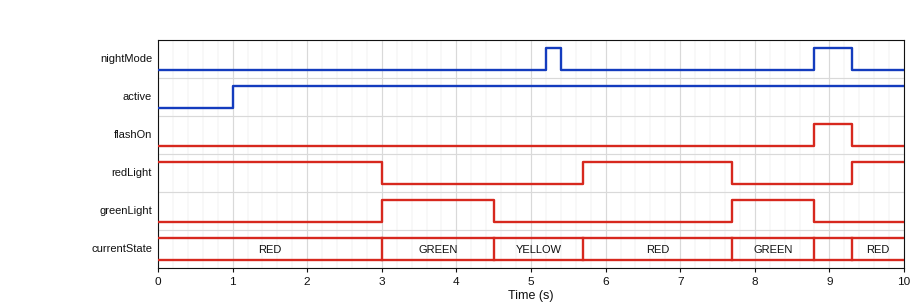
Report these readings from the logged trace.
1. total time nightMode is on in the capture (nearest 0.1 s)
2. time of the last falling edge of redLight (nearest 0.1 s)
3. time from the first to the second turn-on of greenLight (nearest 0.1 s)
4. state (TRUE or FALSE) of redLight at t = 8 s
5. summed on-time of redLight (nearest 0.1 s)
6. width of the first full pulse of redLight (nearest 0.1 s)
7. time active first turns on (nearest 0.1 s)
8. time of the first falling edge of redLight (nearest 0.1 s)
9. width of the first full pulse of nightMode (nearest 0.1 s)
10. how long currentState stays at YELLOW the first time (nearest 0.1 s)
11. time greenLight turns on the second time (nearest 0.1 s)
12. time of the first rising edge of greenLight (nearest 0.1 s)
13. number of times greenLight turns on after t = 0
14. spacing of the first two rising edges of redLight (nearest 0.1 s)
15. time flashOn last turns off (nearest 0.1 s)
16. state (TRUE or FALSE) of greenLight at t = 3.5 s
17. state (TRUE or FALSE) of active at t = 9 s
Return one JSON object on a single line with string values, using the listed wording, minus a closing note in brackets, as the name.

{"total time nightMode is on in the capture": "0.7 s", "time of the last falling edge of redLight": "7.7 s", "time from the first to the second turn-on of greenLight": "4.7 s", "state (TRUE or FALSE) of redLight at t = 8 s": "FALSE", "summed on-time of redLight": "5.7 s", "width of the first full pulse of redLight": "2.0 s", "time active first turns on": "1.0 s", "time of the first falling edge of redLight": "3.0 s", "width of the first full pulse of nightMode": "0.2 s", "how long currentState stays at YELLOW the first time": "1.2 s", "time greenLight turns on the second time": "7.7 s", "time of the first rising edge of greenLight": "3.0 s", "number of times greenLight turns on after t = 0": "2", "spacing of the first two rising edges of redLight": "3.6 s", "time flashOn last turns off": "9.3 s", "state (TRUE or FALSE) of greenLight at t = 3.5 s": "TRUE", "state (TRUE or FALSE) of active at t = 9 s": "TRUE"}
